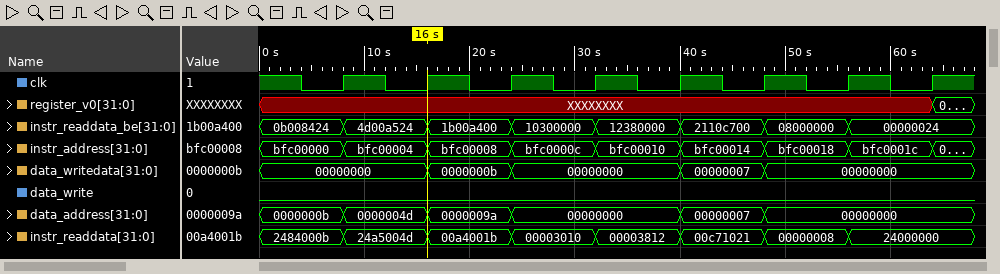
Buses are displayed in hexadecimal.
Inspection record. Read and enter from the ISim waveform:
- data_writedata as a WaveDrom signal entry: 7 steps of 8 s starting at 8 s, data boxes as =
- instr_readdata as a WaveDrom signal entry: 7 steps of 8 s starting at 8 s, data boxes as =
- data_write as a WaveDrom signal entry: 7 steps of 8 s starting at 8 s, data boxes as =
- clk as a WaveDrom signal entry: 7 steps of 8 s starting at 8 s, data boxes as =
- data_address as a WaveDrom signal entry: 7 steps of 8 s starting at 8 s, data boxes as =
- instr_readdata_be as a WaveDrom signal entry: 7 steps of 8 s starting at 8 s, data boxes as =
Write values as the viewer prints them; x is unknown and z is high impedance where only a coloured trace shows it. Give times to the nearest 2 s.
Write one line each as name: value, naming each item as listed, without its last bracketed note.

data_writedata as a WaveDrom signal entry: 7 steps of 8 s starting at 8 s, data boxes as =: {name: 'data_writedata', wave: '===.==.', data: '00000000 0000000b 00000000 00000007 00000000'}
instr_readdata as a WaveDrom signal entry: 7 steps of 8 s starting at 8 s, data boxes as =: {name: 'instr_readdata', wave: '=======', data: '24a5004d 00a4001b 00003010 00003812 00c71021 00000008 24000000'}
data_write as a WaveDrom signal entry: 7 steps of 8 s starting at 8 s, data boxes as =: {name: 'data_write', wave: '0......'}
clk as a WaveDrom signal entry: 7 steps of 8 s starting at 8 s, data boxes as =: {name: 'clk', wave: 'p......'}
data_address as a WaveDrom signal entry: 7 steps of 8 s starting at 8 s, data boxes as =: {name: 'data_address', wave: '===.==.', data: '0000004d 0000009a 00000000 00000007 00000000'}
instr_readdata_be as a WaveDrom signal entry: 7 steps of 8 s starting at 8 s, data boxes as =: {name: 'instr_readdata_be', wave: '=======', data: '4d00a524 1b00a400 10300000 12380000 2110c700 08000000 00000024'}
